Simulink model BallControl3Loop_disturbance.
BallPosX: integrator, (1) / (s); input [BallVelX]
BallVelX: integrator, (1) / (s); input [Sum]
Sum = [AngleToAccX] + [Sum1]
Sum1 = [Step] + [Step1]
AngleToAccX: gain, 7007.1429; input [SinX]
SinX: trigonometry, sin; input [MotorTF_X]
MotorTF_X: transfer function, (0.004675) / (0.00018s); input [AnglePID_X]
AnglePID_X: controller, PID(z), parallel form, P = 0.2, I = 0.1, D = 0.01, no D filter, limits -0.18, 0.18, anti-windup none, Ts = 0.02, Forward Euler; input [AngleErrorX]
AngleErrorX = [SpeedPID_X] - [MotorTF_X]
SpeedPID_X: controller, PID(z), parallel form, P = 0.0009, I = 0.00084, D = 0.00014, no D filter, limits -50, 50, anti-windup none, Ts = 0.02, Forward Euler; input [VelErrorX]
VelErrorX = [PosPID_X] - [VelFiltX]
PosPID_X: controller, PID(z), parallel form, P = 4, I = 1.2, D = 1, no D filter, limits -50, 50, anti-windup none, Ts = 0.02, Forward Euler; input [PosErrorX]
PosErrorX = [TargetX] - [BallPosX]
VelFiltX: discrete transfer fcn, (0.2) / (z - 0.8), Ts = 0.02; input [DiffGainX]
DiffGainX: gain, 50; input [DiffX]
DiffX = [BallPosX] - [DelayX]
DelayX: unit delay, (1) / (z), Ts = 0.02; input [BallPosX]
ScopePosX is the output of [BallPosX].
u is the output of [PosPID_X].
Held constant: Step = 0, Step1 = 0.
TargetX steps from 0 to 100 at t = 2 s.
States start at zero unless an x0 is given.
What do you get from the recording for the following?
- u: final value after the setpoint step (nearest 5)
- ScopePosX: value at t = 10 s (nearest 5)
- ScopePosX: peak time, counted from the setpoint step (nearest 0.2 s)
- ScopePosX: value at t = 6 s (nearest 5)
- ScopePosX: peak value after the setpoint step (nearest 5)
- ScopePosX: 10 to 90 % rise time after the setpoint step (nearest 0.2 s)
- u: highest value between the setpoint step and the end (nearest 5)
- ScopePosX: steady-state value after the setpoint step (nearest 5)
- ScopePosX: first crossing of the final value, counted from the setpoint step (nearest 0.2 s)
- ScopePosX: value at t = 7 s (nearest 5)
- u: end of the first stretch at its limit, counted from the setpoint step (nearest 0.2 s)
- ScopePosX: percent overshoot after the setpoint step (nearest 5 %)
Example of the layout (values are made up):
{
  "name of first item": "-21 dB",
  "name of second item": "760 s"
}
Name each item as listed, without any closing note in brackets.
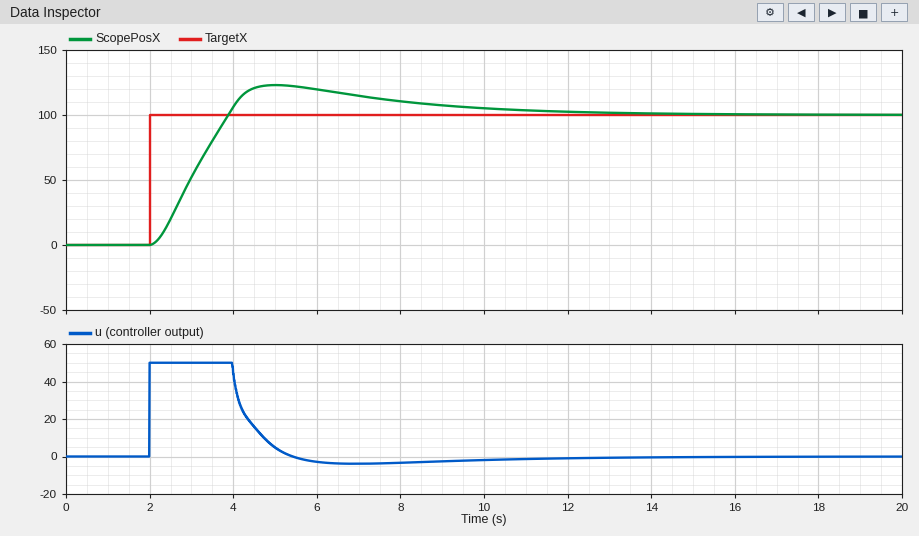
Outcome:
{
  "u: final value after the setpoint step": "0",
  "ScopePosX: value at t = 10 s": "105",
  "ScopePosX: peak time, counted from the setpoint step": "3.0 s",
  "ScopePosX: value at t = 6 s": "120",
  "ScopePosX: peak value after the setpoint step": "125",
  "ScopePosX: 10 to 90 % rise time after the setpoint step": "1.4 s",
  "u: highest value between the setpoint step and the end": "50",
  "ScopePosX: steady-state value after the setpoint step": "100",
  "ScopePosX: first crossing of the final value, counted from the setpoint step": "1.8 s",
  "ScopePosX: value at t = 7 s": "115",
  "u: end of the first stretch at its limit, counted from the setpoint step": "2.0 s",
  "ScopePosX: percent overshoot after the setpoint step": "25 %"
}
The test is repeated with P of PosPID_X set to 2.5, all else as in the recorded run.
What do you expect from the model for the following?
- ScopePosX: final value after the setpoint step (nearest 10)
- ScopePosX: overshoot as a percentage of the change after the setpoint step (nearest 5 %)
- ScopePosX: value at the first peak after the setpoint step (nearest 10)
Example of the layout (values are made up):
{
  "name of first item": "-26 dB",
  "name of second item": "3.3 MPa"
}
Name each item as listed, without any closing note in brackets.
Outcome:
{
  "ScopePosX: final value after the setpoint step": "100",
  "ScopePosX: overshoot as a percentage of the change after the setpoint step": "30 %",
  "ScopePosX: value at the first peak after the setpoint step": "130"
}
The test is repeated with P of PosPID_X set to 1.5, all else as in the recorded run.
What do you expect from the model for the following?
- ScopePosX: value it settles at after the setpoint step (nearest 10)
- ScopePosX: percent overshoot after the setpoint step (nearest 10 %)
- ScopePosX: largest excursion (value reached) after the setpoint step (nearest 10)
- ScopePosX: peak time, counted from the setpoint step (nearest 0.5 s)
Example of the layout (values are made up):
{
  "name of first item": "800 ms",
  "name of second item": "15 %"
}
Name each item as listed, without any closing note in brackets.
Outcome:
{
  "ScopePosX: value it settles at after the setpoint step": "100",
  "ScopePosX: percent overshoot after the setpoint step": "40 %",
  "ScopePosX: largest excursion (value reached) after the setpoint step": "140",
  "ScopePosX: peak time, counted from the setpoint step": "3.5 s"
}
